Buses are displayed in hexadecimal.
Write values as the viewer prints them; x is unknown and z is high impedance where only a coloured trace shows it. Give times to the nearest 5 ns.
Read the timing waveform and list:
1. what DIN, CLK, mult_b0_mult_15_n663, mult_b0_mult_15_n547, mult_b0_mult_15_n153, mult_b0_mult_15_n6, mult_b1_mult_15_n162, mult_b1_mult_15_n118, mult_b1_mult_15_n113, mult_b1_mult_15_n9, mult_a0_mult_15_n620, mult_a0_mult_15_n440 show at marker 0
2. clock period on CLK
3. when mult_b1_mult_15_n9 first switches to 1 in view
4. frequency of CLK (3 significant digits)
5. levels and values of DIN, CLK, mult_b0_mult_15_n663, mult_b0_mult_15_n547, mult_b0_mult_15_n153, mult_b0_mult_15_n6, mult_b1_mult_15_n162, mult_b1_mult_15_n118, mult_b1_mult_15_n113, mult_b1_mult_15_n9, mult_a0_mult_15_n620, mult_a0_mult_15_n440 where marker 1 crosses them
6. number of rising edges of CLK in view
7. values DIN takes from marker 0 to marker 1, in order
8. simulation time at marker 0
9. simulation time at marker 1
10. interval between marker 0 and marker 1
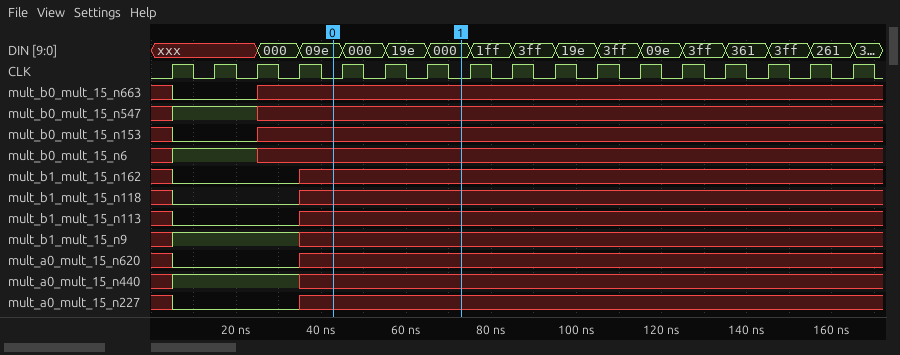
DIN=09e, CLK=0, mult_b0_mult_15_n663=x, mult_b0_mult_15_n547=x, mult_b0_mult_15_n153=x, mult_b0_mult_15_n6=x, mult_b1_mult_15_n162=x, mult_b1_mult_15_n118=x, mult_b1_mult_15_n113=x, mult_b1_mult_15_n9=x, mult_a0_mult_15_n620=x, mult_a0_mult_15_n440=x
10 ns
5 ns
100 MHz
DIN=000, CLK=0, mult_b0_mult_15_n663=x, mult_b0_mult_15_n547=x, mult_b0_mult_15_n153=x, mult_b0_mult_15_n6=x, mult_b1_mult_15_n162=x, mult_b1_mult_15_n118=x, mult_b1_mult_15_n113=x, mult_b1_mult_15_n9=x, mult_a0_mult_15_n620=x, mult_a0_mult_15_n440=x
17
09e, 000, 19e, 000
45 ns
75 ns
30 ns
